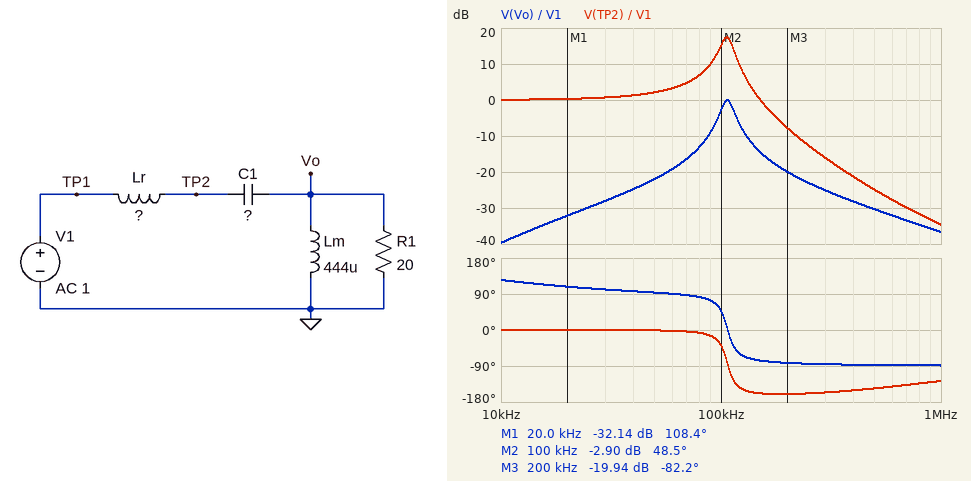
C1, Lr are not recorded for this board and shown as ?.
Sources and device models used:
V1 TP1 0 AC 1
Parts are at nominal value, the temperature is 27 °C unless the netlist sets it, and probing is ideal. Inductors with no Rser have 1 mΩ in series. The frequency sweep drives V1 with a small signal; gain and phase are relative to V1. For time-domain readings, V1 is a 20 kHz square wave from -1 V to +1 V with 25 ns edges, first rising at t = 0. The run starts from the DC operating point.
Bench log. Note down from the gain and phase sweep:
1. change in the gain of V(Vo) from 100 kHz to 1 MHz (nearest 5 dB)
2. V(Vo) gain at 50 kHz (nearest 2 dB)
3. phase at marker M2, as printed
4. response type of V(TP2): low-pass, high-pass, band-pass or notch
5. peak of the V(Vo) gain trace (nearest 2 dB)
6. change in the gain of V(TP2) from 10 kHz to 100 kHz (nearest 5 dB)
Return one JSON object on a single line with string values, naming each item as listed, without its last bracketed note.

{"change in the gain of V(Vo) from 100 kHz to 1 MHz": "-35 dB", "V(Vo) gain at 50 kHz": "-22 dB", "phase at marker M2, as printed": "48.5 deg", "response type of V(TP2): low-pass, high-pass, band-pass or notch": "low-pass", "peak of the V(Vo) gain trace": "0 dB", "change in the gain of V(TP2) from 10 kHz to 100 kHz": "15 dB"}
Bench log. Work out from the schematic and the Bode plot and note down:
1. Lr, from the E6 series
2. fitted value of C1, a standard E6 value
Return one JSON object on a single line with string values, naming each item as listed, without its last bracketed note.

{"Lr, from the E6 series": "220 µH", "fitted value of C1, a standard E6 value": "10 nF"}
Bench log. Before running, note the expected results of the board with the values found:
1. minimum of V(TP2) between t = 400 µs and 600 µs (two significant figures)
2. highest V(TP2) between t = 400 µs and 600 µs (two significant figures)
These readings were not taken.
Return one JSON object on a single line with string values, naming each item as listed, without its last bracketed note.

{"minimum of V(TP2) between t = 400 µs and 600 µs": "-2.9 V", "highest V(TP2) between t = 400 µs and 600 µs": "2.9 V"}
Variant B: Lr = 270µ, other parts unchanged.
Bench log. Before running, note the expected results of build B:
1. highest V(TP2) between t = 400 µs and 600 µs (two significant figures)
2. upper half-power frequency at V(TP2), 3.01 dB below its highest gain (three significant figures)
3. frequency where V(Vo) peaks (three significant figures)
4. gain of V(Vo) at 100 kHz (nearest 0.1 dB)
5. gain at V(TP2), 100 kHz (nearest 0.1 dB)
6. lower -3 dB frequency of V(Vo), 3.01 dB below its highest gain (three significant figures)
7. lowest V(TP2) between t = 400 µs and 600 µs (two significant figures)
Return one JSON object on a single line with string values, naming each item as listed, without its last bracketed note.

{"highest V(TP2) between t = 400 µs and 600 µs": "3.3 V", "upper half-power frequency at V(TP2), 3.01 dB below its highest gain": "102 kHz", "frequency where V(Vo) peaks": "96.4 kHz", "gain of V(Vo) at 100 kHz": "-1.3 dB", "gain at V(TP2), 100 kHz": "16.7 dB", "lower -3 dB frequency of V(Vo), 3.01 dB below its highest gain": "90.7 kHz", "lowest V(TP2) between t = 400 µs and 600 µs": "-3.3 V"}
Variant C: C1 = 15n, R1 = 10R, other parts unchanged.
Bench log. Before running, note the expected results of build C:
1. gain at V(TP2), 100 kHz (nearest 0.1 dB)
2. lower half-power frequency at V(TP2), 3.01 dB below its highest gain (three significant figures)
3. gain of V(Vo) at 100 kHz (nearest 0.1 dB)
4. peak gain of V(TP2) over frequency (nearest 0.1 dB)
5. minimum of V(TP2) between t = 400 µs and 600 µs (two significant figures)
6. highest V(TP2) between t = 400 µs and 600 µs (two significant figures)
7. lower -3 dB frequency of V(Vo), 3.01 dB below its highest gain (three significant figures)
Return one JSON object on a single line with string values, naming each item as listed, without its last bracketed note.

{"gain at V(TP2), 100 kHz": "9.9 dB", "lower half-power frequency at V(TP2), 3.01 dB below its highest gain": "83.6 kHz", "gain of V(Vo) at 100 kHz": "-10.6 dB", "peak gain of V(TP2) over frequency": "21.7 dB", "minimum of V(TP2) between t = 400 µs and 600 µs": "-2.3 V", "highest V(TP2) between t = 400 µs and 600 µs": "2.3 V", "lower -3 dB frequency of V(Vo), 3.01 dB below its highest gain": "83.9 kHz"}
